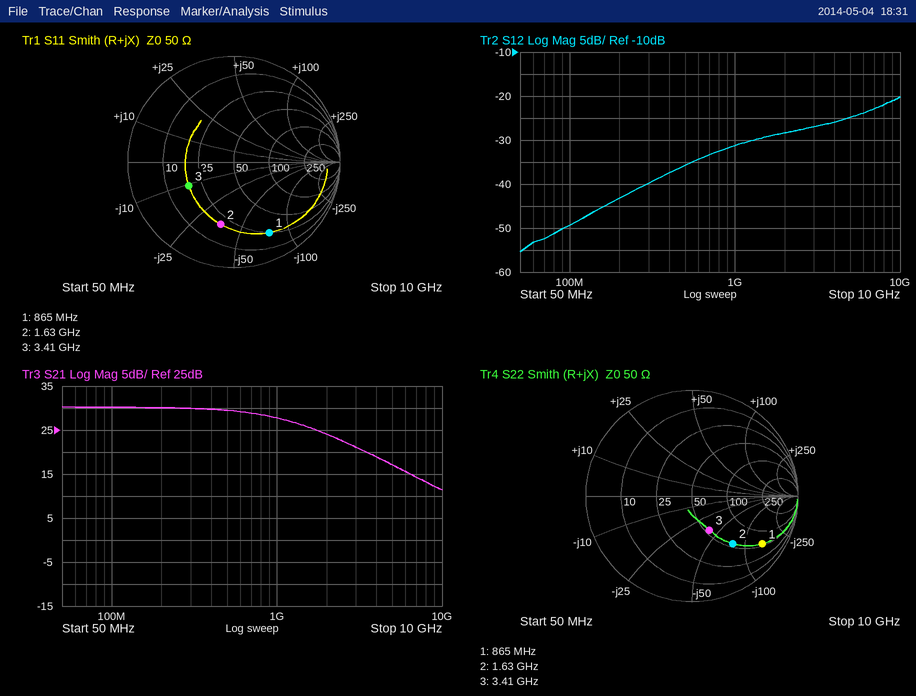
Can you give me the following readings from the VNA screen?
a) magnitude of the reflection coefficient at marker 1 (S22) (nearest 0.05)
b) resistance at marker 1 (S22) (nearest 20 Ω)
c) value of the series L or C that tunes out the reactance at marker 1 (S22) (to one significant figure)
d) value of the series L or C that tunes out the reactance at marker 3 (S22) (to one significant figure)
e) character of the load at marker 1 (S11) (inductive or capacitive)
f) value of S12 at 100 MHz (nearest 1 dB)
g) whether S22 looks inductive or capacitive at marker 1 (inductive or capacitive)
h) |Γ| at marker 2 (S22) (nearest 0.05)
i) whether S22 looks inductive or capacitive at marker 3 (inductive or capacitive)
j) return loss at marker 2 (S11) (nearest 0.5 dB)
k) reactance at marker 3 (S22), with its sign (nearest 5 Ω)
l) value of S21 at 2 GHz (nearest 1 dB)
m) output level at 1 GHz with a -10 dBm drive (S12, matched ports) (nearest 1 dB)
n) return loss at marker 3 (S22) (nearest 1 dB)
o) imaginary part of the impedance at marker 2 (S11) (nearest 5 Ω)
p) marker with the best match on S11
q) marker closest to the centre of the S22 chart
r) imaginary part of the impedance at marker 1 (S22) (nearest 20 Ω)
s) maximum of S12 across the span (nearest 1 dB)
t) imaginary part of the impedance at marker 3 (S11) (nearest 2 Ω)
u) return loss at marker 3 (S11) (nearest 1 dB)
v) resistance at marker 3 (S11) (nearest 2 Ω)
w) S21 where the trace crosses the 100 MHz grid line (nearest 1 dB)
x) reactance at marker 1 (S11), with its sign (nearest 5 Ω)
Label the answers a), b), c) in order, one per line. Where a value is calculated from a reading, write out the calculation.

a) 0.80
b) 60 Ω
c) L = 140 Ω/(2π × 865 MHz) ≈ 25.8 nH, so 30 nH to one significant figure
d) L = 40 Ω/(2π × 3.41 GHz) ≈ 2 nH
e) capacitive
f) -49 dB
g) capacitive
h) 0.60
i) capacitive
j) 4.5 dB
k) -40 Ω
l) 24 dB
m) -10 dBm + (-31 dB) = -41 dBm
n) 9 dB
o) -35 Ω
p) marker 3
q) marker 3
r) -140 Ω
s) -20 dB
t) -10 Ω
u) 6 dB
v) 18 Ω
w) 30 dB
x) -75 Ω
